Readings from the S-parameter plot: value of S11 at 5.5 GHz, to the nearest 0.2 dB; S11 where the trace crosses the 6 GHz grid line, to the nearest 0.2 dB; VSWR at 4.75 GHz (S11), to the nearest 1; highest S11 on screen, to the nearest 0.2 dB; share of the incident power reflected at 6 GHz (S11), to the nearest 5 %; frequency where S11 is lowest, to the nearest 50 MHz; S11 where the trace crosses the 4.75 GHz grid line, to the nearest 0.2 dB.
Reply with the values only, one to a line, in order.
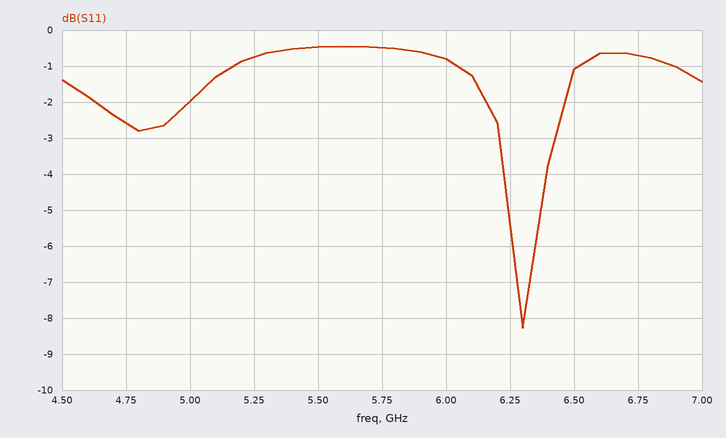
-0.4 dB
-0.8 dB
7
-0.4 dB
85 %
6.30 GHz
-2.6 dB
